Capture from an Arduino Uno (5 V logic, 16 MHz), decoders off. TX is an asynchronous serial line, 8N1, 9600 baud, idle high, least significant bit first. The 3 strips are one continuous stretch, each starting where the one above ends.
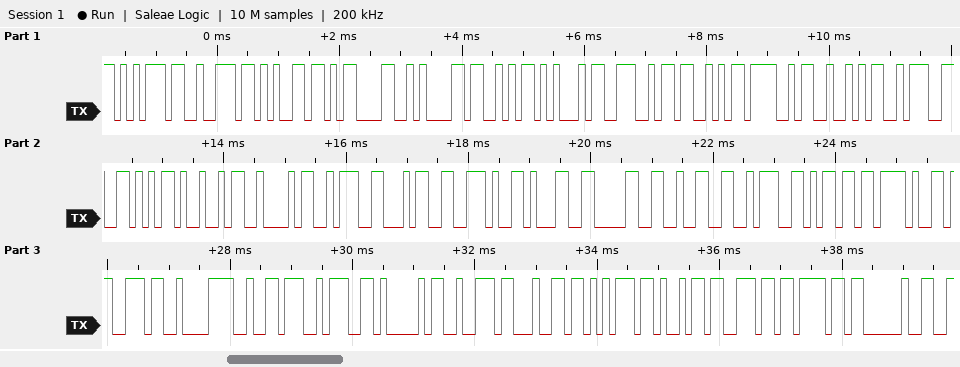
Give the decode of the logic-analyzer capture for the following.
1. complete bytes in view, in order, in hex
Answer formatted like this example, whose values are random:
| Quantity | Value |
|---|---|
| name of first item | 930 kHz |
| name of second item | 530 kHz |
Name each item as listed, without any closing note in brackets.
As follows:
| Quantity | Value |
|---|---|
| complete bytes in view, in order, in hex | 75 72 65 0D 0A 53 45 4E 53 4F 52 3A 56 49 42 3A 34 2E 31 30 32 3A 6D 2F 73 C2 B2 3A 41 72 64 75 69 6E 6F 20 |
